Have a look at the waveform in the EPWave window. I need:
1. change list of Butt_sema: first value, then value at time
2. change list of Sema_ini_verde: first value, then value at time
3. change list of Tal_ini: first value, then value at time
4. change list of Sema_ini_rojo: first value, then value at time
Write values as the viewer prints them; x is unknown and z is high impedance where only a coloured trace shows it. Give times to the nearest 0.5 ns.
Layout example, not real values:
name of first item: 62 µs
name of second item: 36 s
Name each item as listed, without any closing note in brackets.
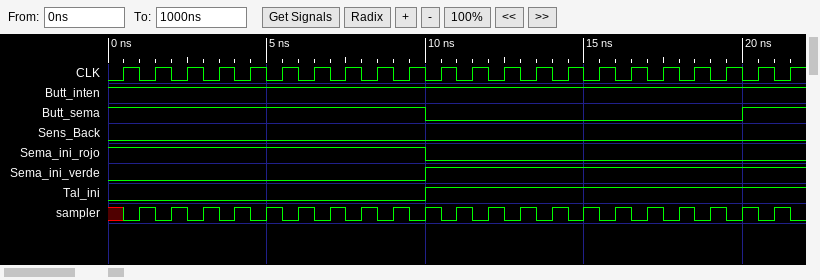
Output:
change list of Butt_sema: first value, then value at time: 1, 0 at 10 ns, 1 at 20 ns
change list of Sema_ini_verde: first value, then value at time: 0, 1 at 10 ns
change list of Tal_ini: first value, then value at time: 0, 1 at 10 ns
change list of Sema_ini_rojo: first value, then value at time: 1, 0 at 10 ns
